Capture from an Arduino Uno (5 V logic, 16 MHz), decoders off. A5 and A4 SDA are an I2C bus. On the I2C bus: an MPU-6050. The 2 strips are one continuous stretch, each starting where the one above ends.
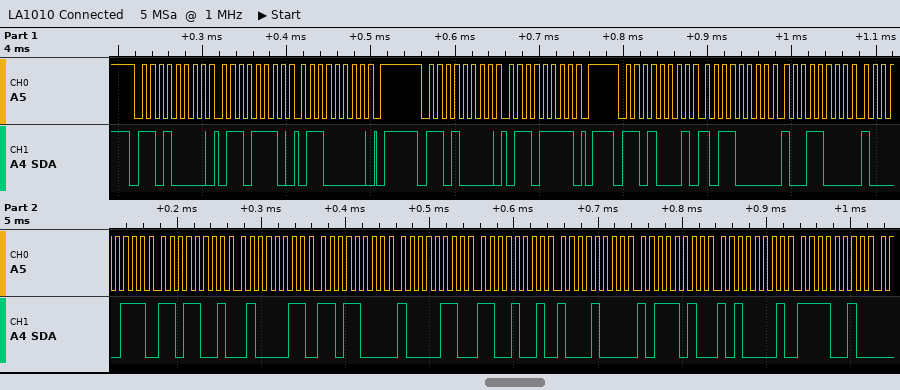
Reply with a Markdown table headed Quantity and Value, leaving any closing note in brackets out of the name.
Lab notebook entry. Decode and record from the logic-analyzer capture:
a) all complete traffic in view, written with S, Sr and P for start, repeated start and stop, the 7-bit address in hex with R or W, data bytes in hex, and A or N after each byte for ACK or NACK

| Quantity | Value |
|---|---|
| all complete traffic in view, written with S, Sr and P for start, repeated start and stop, the 7-bit address in hex with R or W, data bytes in hex, and A or N after each byte for ACK or NACK | S 68W A 6E A 60 A P S 68W A 6F A P S 68R A B0 A 98 A 87 A D9 A 43 A D8 A 86 A C9 A 88 A BA A A1 A F2 A |
